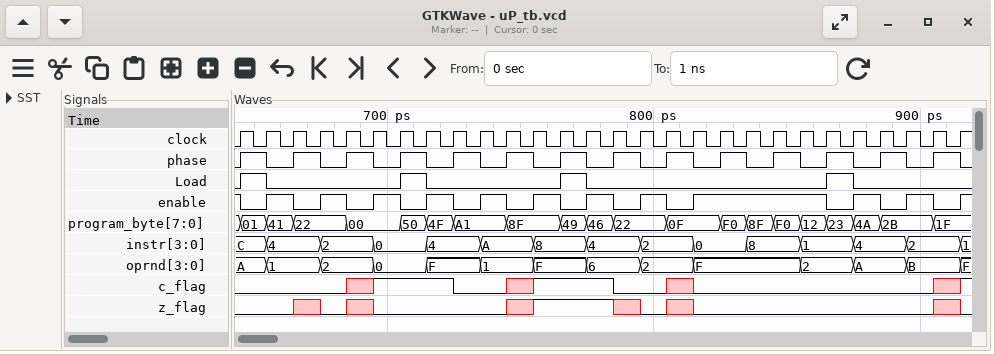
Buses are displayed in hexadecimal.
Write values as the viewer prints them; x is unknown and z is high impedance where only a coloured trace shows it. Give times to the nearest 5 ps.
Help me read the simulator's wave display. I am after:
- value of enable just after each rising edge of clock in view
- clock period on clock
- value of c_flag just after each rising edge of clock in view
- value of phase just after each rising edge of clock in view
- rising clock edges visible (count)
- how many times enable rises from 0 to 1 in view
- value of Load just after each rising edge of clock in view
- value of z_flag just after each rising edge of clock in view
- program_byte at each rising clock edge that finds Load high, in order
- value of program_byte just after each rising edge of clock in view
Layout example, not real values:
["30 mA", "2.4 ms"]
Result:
["0 1 0 1 0 1 0 1 0 1 0 1 0 1 0 1 0 1 1 1 1 1 0 1 0 1 0 1", "10 ps", "0 0 0 0 x 1 1 1 0 0 x 1 1 1 0 0 x 0 0 0 0 0 0 0 0 0 x 1", "1 0 1 0 1 0 1 0 1 0 1 0 1 0 1 0 1 0 1 0 1 0 1 0 1 0 1 0", "28", "12", "1 0 0 0 0 0 1 0 0 0 0 0 1 0 0 0 0 0 0 0 0 0 1 0 0 0 0 0", "0 0 x 0 x 0 0 0 0 0 x 1 1 1 x 0 x 0 0 0 0 0 0 0 0 0 x 0", "01, 50, 49, 23", "01, 41, 22, 22, 00, 00, 50, 4F, A1, A1, 8F, 8F, 49, 46, 22, 22, 0F, 0F, F0, 8F, F0, 12, 23, 4A, 2B, 2B, 1F, 1F"]
